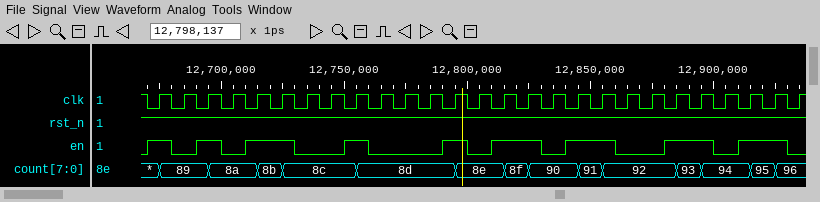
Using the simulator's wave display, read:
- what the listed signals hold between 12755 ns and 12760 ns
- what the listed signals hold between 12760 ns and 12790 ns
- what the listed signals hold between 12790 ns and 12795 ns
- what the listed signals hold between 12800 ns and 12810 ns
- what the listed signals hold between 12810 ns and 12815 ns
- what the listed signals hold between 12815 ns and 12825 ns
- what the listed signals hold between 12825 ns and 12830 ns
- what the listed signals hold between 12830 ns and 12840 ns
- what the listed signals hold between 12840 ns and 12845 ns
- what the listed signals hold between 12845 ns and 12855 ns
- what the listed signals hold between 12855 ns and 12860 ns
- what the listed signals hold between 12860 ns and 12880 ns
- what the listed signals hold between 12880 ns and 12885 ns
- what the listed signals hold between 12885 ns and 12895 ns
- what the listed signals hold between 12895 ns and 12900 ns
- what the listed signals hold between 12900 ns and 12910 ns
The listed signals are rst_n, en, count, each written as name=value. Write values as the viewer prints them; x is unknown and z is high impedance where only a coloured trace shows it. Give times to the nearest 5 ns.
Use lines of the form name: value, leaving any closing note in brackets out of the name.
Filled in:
what the listed signals hold between 12755 ns and 12760 ns: rst_n=1, en=1, count=8d
what the listed signals hold between 12760 ns and 12790 ns: rst_n=1, en=0, count=8d
what the listed signals hold between 12790 ns and 12795 ns: rst_n=1, en=1, count=8d
what the listed signals hold between 12800 ns and 12810 ns: rst_n=1, en=0, count=8e
what the listed signals hold between 12810 ns and 12815 ns: rst_n=1, en=1, count=8e
what the listed signals hold between 12815 ns and 12825 ns: rst_n=1, en=1, count=8f
what the listed signals hold between 12825 ns and 12830 ns: rst_n=1, en=1, count=90
what the listed signals hold between 12830 ns and 12840 ns: rst_n=1, en=0, count=90
what the listed signals hold between 12840 ns and 12845 ns: rst_n=1, en=1, count=90
what the listed signals hold between 12845 ns and 12855 ns: rst_n=1, en=1, count=91
what the listed signals hold between 12855 ns and 12860 ns: rst_n=1, en=1, count=92
what the listed signals hold between 12860 ns and 12880 ns: rst_n=1, en=0, count=92
what the listed signals hold between 12880 ns and 12885 ns: rst_n=1, en=1, count=92
what the listed signals hold between 12885 ns and 12895 ns: rst_n=1, en=1, count=93
what the listed signals hold between 12895 ns and 12900 ns: rst_n=1, en=1, count=94
what the listed signals hold between 12900 ns and 12910 ns: rst_n=1, en=0, count=94
